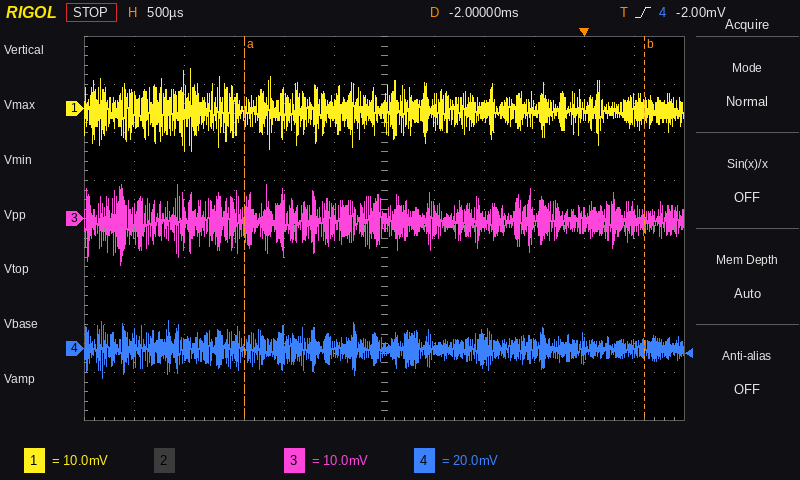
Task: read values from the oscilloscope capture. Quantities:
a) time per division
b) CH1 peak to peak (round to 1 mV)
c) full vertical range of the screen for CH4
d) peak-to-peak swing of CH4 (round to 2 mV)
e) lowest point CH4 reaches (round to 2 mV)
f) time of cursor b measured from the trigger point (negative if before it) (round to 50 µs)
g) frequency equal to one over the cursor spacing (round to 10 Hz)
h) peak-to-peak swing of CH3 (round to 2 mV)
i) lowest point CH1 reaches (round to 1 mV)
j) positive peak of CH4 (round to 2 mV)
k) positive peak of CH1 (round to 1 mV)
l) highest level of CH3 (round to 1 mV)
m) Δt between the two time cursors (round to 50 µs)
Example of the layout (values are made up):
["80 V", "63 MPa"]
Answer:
["500 µs", "17 mV", "160 mV", "24 mV", "-12 mV", "+600 µs", "250 Hz", "16 mV", "-9 mV", "12 mV", "8 mV", "7 mV", "4.00 ms"]
